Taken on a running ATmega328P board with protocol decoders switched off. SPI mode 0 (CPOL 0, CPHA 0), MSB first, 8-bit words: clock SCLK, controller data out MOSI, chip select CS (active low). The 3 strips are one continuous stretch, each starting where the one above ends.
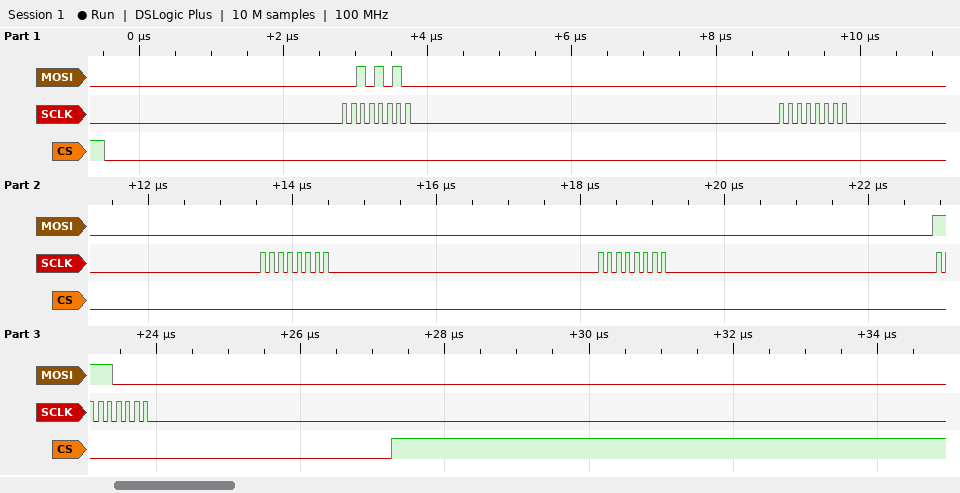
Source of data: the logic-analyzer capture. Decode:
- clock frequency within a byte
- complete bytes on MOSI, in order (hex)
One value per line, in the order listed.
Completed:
8 MHz
2A 00 00 00 F0
